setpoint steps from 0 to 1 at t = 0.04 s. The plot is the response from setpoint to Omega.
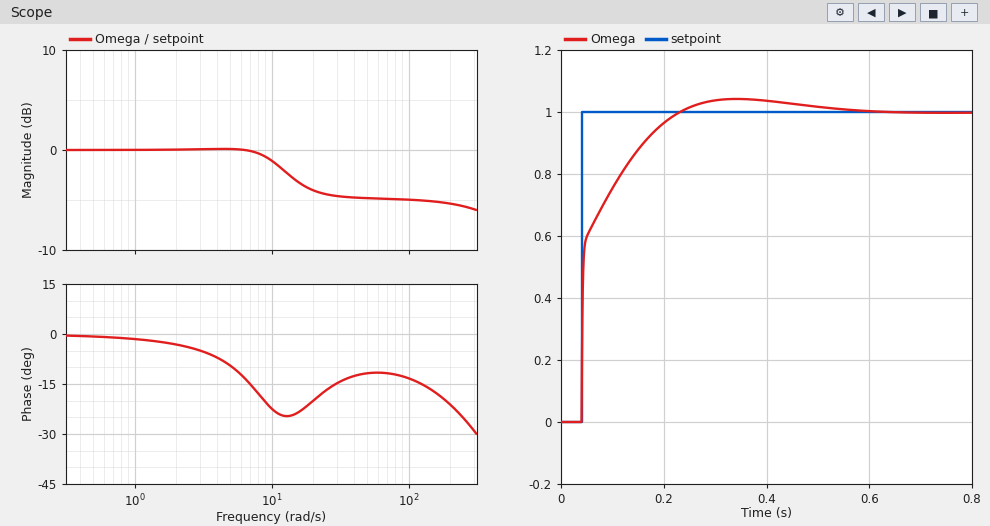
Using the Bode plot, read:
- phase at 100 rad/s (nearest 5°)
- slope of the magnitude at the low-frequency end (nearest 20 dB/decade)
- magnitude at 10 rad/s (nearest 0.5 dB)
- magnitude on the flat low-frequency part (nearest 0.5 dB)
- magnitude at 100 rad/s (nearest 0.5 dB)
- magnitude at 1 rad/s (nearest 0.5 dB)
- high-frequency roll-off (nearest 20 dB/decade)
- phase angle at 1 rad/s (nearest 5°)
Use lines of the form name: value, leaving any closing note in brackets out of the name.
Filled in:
phase at 100 rad/s: -15°
slope of the magnitude at the low-frequency end: 0 dB/decade
magnitude at 10 rad/s: -1.0 dB
magnitude on the flat low-frequency part: 0.0 dB
magnitude at 100 rad/s: -5.0 dB
magnitude at 1 rad/s: 0.0 dB
high-frequency roll-off: 0 dB/decade
phase angle at 1 rad/s: 0°
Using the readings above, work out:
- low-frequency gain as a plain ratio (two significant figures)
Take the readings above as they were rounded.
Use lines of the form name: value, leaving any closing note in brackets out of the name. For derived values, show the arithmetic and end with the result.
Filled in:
low-frequency gain as a plain ratio: 10^(0 / 20) = 1.0
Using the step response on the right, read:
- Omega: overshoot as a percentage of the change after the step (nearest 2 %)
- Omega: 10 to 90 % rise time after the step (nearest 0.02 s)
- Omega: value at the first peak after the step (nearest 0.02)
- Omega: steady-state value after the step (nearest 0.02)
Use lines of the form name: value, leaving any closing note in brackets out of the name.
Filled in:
Omega: overshoot as a percentage of the change after the step: 4 %
Omega: 10 to 90 % rise time after the step: 0.12 s
Omega: value at the first peak after the step: 1.04
Omega: steady-state value after the step: 1.00
